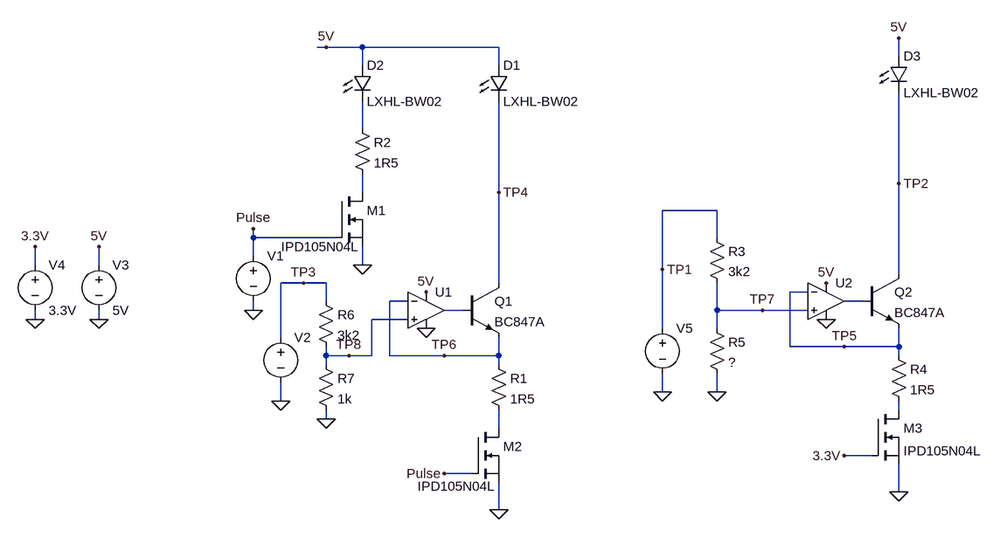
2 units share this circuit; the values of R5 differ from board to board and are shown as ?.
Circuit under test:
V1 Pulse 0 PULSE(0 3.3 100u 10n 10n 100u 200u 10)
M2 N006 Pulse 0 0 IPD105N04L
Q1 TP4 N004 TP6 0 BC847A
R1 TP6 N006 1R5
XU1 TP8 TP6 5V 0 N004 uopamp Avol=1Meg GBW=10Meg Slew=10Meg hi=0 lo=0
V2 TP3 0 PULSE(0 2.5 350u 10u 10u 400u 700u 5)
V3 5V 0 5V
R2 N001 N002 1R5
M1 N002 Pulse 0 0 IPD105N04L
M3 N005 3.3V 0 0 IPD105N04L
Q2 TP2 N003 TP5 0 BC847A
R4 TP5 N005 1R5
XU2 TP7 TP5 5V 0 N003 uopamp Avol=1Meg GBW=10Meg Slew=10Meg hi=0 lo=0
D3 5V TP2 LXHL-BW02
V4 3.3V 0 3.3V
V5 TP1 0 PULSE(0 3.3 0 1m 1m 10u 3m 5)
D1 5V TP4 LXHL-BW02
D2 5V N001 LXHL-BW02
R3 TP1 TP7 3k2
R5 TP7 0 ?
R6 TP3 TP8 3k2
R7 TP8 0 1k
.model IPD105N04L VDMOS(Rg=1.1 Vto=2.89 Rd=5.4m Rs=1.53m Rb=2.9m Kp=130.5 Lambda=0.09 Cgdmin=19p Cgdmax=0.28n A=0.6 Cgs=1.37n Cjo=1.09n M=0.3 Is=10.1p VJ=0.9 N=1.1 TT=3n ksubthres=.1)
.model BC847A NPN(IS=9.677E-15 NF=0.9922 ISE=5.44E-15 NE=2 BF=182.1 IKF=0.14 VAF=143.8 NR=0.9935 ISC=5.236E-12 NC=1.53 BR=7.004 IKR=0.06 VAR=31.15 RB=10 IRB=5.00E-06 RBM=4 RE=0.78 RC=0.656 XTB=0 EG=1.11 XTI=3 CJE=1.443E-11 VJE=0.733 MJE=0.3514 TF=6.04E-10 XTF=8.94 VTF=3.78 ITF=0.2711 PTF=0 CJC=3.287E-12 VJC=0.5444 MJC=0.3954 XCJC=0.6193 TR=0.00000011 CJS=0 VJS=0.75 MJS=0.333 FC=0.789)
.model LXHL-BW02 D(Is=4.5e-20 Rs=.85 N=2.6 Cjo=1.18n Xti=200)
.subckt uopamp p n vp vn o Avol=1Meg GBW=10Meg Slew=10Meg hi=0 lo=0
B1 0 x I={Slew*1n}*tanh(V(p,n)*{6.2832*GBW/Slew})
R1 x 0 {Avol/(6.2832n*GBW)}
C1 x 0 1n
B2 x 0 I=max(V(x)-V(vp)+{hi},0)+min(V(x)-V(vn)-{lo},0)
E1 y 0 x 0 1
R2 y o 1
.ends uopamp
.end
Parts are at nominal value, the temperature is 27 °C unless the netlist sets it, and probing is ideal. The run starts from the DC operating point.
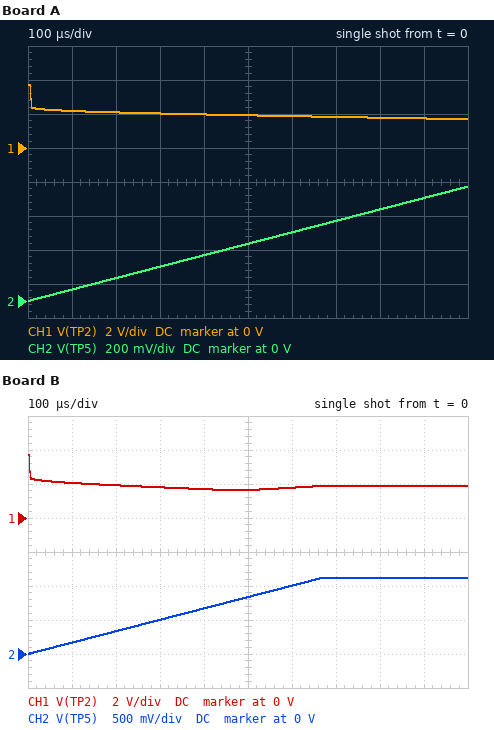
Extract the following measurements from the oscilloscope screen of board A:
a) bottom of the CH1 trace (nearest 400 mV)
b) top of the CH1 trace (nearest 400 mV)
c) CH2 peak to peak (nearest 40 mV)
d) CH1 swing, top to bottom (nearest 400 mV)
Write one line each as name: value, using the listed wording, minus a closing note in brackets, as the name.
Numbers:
bottom of the CH1 trace: 1.6 V
top of the CH1 trace: 3.6 V
CH2 peak to peak: 680 mV
CH1 swing, top to bottom: 2.0 V
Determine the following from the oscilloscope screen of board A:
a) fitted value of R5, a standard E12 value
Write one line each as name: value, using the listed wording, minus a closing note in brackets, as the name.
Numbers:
fitted value of R5, a standard E12 value: 820 Ω
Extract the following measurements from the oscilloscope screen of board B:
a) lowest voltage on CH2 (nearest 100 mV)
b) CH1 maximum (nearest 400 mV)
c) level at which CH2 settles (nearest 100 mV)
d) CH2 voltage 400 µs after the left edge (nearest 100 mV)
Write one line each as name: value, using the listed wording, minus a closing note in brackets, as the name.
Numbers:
lowest voltage on CH2: 0 V
CH1 maximum: 3.6 V
level at which CH2 settles: 1.1 V
CH2 voltage 400 µs after the left edge: 700 mV
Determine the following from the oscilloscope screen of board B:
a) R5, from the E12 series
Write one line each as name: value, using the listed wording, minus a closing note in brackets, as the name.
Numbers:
R5, from the E12 series: 3.3 kΩ
